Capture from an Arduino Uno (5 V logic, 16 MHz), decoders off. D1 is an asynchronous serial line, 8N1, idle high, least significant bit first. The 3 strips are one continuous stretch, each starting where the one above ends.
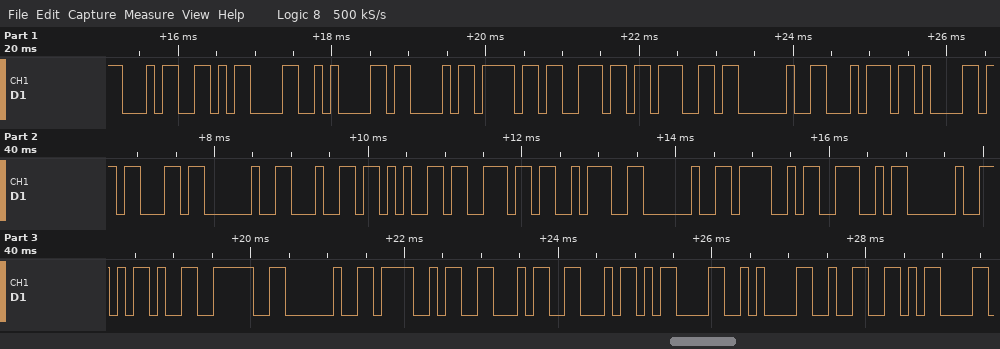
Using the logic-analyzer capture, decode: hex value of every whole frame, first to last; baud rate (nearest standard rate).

0x34 0x0D 0x0A 0x43 0x6F 0x6E 0x67 0x20 0x74 0x61 0x63 0x20 0x64 0x65 0x6E 0x3A 0x20 0x4F 0x4E 0x20 0x2D 0x3E 0x20 0x4F 0x46 0x46 0x0D 0x0A 0x32 0x0D
9600 baud
